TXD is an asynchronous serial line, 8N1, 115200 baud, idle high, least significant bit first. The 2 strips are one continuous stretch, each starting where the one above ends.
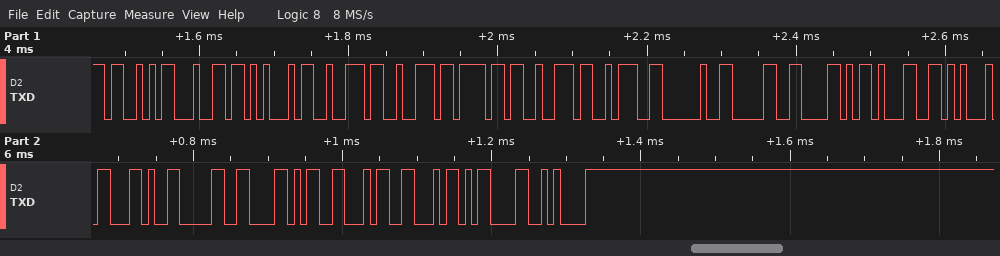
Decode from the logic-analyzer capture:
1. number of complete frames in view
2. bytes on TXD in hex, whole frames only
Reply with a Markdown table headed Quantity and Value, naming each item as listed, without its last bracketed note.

| Quantity | Value |
|---|---|
| number of complete frames in view | 20 |
| bytes on TXD in hex, whole frames only | 0x53 0x64 0x45 0x72 0x72 0x6F 0x72 0x3A 0x20 0x30 0x58 0x31 0x45 0x2C 0x30 0x58 0x46 0x46 0x0D 0x0A |
